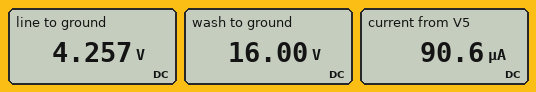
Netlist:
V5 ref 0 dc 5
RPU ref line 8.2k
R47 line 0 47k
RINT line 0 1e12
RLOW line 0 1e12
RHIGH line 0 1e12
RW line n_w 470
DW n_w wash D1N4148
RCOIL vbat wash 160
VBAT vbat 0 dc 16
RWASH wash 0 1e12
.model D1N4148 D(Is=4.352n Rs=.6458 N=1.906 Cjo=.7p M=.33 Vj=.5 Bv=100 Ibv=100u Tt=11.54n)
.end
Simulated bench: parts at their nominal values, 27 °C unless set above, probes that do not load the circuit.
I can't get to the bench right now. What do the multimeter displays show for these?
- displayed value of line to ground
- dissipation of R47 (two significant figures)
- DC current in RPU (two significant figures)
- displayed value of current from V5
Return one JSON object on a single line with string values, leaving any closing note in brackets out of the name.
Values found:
{"displayed value of line to ground": "4.257 V", "dissipation of R47": "390 µW", "DC current in RPU": "91 µA", "displayed value of current from V5": "90.6 µA"}
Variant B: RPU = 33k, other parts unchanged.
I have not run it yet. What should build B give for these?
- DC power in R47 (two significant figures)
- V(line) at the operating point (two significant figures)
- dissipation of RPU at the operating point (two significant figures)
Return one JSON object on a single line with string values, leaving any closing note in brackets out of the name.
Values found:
{"DC power in R47": "180 µW", "V(line) at the operating point": "2.9 V", "dissipation of RPU at the operating point": "130 µW"}
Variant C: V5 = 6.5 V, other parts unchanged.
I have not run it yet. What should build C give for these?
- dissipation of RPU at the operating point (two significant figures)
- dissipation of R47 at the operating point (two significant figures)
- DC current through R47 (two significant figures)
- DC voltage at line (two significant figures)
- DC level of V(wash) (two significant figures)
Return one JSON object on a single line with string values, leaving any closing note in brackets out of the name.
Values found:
{"dissipation of RPU at the operating point": "110 µW", "dissipation of R47 at the operating point": "650 µW", "DC current through R47": "120 µA", "DC voltage at line": "5.5 V", "DC level of V(wash)": "16 V"}
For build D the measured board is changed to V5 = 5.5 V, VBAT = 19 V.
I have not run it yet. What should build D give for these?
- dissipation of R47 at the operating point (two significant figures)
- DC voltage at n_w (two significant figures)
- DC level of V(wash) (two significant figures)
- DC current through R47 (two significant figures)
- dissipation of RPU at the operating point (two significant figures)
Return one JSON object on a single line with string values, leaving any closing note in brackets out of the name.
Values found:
{"dissipation of R47 at the operating point": "470 µW", "DC voltage at n_w": "4.7 V", "DC level of V(wash)": "19 V", "DC current through R47": "100 µA", "dissipation of RPU at the operating point": "81 µW"}
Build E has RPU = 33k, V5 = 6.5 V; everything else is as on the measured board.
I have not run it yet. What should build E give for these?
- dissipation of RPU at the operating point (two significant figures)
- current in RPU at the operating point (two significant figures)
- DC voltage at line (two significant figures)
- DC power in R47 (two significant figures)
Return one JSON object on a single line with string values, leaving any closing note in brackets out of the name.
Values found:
{"dissipation of RPU at the operating point": "220 µW", "current in RPU at the operating point": "81 µA", "DC voltage at line": "3.8 V", "DC power in R47": "310 µW"}
